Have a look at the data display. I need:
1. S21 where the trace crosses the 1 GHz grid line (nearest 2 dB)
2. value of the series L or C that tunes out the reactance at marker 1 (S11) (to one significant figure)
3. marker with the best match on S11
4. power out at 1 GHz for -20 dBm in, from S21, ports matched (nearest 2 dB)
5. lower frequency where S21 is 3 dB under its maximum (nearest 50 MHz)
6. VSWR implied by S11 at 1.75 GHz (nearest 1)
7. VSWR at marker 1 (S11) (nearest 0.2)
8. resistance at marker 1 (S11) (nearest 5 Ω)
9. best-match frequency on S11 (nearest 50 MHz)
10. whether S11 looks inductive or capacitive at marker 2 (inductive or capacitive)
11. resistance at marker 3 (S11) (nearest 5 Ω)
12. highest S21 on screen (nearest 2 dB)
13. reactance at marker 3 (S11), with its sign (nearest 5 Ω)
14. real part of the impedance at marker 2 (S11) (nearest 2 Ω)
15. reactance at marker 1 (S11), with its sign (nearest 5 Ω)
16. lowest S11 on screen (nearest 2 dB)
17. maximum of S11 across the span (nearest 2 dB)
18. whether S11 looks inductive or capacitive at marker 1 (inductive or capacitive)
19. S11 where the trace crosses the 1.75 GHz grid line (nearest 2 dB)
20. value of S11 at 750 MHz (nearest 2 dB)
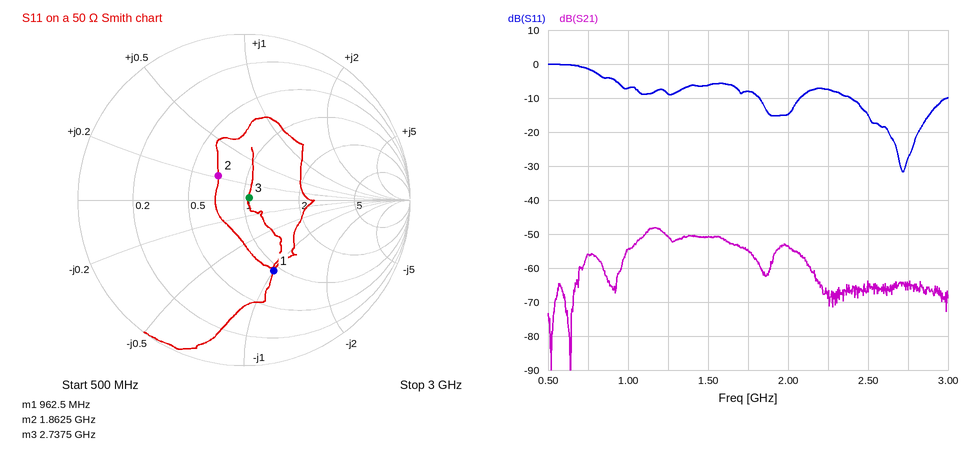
-54 dB
8 nH
marker 3
-74 dBm
1.10 GHz
2
2.8
45 Ω
2.70 GHz
inductive
55 Ω
-48 dB
0 Ω
36 Ω
-50 Ω
-32 dB
0 dB
capacitive
-8 dB
-2 dB
